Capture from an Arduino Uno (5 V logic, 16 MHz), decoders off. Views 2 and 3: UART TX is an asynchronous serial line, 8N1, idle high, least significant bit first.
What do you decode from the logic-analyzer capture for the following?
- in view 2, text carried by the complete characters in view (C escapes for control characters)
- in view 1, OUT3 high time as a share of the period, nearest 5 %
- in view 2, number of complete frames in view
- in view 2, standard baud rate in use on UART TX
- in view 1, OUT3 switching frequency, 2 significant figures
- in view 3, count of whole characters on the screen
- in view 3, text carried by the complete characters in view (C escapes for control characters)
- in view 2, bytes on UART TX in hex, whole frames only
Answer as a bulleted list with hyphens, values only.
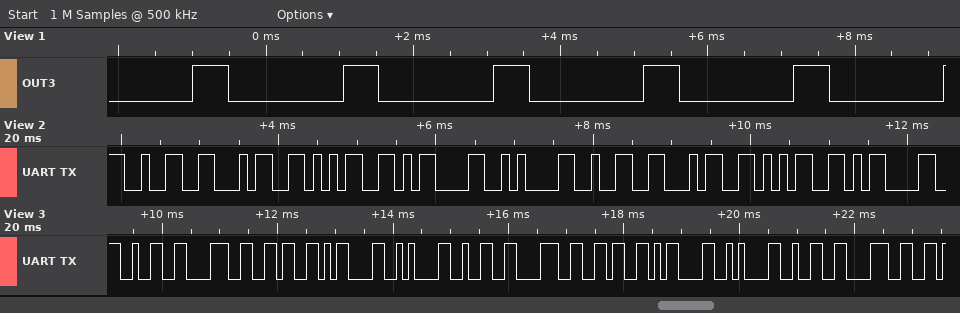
- "245\r\n245\r"
- 25 %
- 9
- 9600 baud
- 490 Hz
- 12
- "286\r\n286\r\n28"
- 0x32 0x34 0x35 0x0D 0x0A 0x32 0x34 0x35 0x0D
